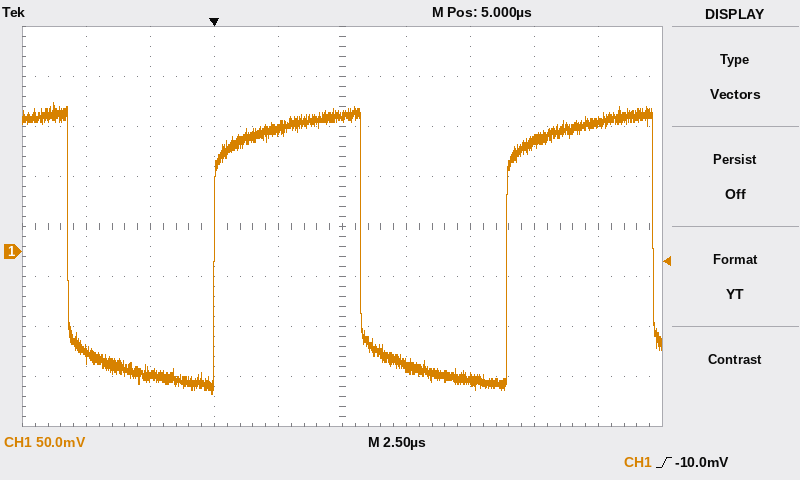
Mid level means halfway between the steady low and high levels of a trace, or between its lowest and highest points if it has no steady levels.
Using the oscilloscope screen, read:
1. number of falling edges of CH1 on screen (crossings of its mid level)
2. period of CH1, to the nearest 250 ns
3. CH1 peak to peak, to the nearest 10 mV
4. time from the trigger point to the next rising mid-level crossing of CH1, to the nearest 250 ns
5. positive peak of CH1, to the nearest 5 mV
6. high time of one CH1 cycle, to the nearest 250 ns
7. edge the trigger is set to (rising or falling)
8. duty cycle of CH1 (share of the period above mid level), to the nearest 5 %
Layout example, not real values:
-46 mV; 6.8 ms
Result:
3; 11.50 µs; 290 mV; 11.50 µs; 150 mV; 5.75 µs; rising; 50 %
